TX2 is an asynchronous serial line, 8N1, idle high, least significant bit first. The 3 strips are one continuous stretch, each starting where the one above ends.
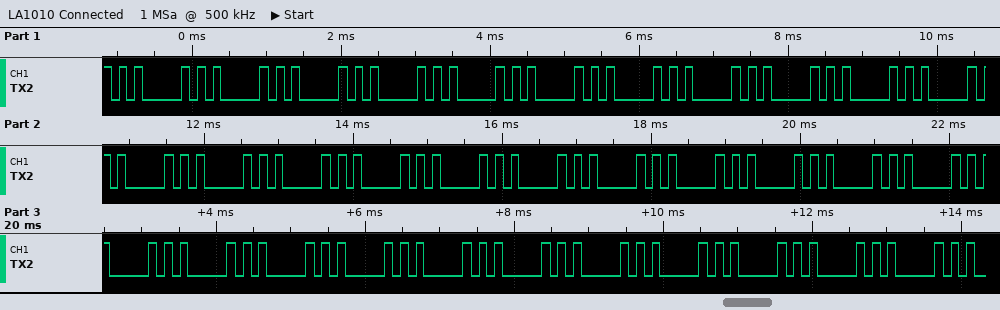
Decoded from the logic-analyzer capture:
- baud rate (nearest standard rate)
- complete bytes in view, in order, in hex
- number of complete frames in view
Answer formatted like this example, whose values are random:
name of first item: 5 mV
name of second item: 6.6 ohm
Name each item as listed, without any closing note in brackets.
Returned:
baud rate: 9600 baud
complete bytes in view, in order, in hex: 05 05 05 05 05 05 05 05 05 05 05 05 05 05 05 05 05 05 05 05 05 05 05 05 05 05 05 05 05 05 05 05 05
number of complete frames in view: 33
